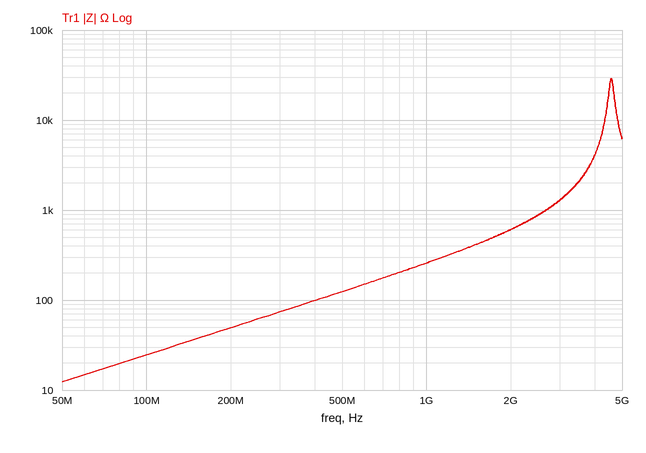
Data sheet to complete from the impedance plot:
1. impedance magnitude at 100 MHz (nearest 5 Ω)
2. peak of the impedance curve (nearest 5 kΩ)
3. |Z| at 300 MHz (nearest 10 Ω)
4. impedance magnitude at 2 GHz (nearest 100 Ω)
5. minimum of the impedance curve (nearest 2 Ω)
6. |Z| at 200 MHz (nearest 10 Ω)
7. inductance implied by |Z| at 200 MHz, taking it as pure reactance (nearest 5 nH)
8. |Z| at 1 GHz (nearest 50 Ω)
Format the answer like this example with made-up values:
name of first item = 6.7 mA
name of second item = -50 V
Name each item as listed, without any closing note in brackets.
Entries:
impedance magnitude at 100 MHz = 25 Ω
peak of the impedance curve = 30 kΩ
|Z| at 300 MHz = 70 Ω
impedance magnitude at 2 GHz = 600 Ω
minimum of the impedance curve = 12 Ω
|Z| at 200 MHz = 50 Ω
inductance implied by |Z| at 200 MHz, taking it as pure reactance = 40 nH
|Z| at 1 GHz = 250 Ω
